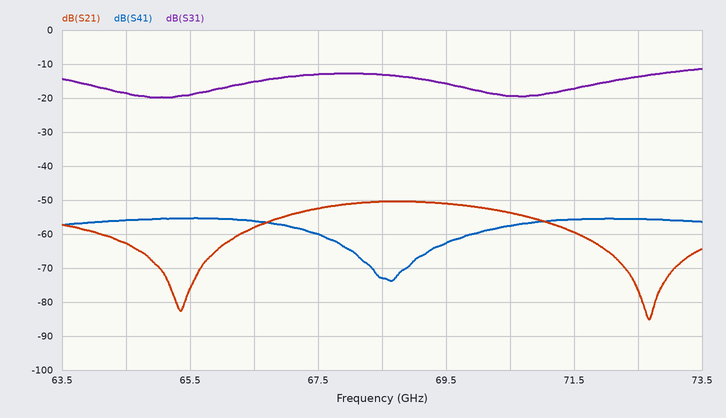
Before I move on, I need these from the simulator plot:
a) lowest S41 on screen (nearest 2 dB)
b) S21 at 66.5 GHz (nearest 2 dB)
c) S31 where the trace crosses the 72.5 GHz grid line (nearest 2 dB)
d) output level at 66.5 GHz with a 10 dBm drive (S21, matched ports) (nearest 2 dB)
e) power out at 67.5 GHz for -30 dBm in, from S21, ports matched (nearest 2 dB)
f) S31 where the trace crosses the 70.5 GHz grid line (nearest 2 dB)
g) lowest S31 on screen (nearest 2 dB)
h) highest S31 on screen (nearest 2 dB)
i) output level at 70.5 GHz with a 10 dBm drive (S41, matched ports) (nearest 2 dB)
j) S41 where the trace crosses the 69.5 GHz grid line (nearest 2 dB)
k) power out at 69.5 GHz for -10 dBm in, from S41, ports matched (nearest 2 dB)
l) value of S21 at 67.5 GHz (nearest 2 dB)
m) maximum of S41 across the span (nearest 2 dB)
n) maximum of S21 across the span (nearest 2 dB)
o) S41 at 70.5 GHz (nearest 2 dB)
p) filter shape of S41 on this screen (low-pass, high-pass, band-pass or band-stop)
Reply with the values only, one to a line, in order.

-74 dB
-58 dB
-14 dB
-48 dBm
-82 dBm
-20 dB
-20 dB
-12 dB
-48 dBm
-62 dB
-72 dBm
-52 dB
-56 dB
-50 dB
-58 dB
band-stop
